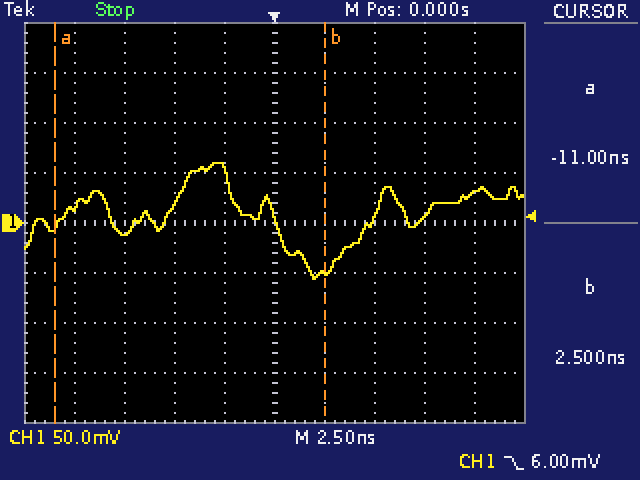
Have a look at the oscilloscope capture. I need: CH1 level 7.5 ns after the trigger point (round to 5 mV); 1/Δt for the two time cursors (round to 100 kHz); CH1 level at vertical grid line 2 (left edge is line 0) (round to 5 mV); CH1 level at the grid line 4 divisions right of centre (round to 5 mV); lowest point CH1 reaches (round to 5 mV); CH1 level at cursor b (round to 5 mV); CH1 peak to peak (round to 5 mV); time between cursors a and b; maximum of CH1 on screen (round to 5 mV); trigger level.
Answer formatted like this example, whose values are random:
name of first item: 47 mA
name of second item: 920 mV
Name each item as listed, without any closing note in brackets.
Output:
CH1 level 7.5 ns after the trigger point: 5 mV
1/Δt for the two time cursors: 74.1 MHz
CH1 level at vertical grid line 2 (left edge is line 0): -10 mV
CH1 level at the grid line 4 divisions right of centre: 30 mV
lowest point CH1 reaches: -55 mV
CH1 level at cursor b: -50 mV
CH1 peak to peak: 115 mV
time between cursors a and b: 13.50 ns
maximum of CH1 on screen: 60 mV
trigger level: 6.00 mV
